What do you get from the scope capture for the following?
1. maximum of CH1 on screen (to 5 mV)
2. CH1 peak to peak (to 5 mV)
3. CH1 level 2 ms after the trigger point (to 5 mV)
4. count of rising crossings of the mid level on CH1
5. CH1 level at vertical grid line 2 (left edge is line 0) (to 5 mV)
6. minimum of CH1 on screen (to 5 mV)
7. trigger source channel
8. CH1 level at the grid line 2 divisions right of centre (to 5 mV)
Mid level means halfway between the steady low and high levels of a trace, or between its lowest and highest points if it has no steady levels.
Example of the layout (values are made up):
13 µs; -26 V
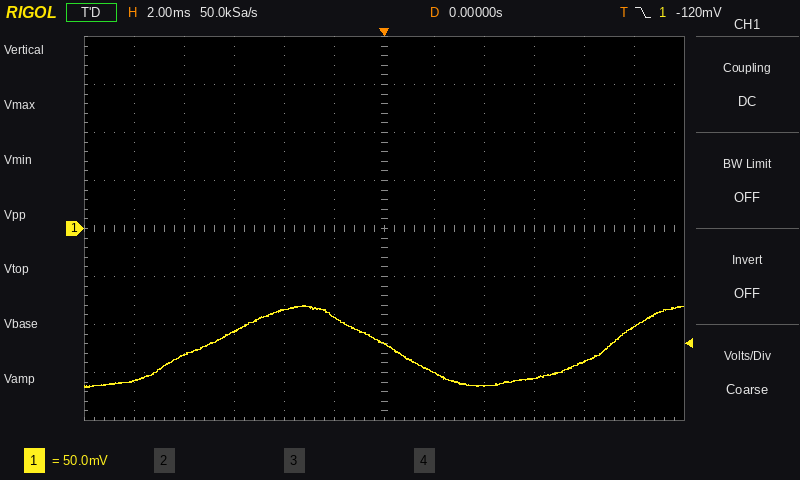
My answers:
-80 mV; 85 mV; -150 mV; 2; -130 mV; -165 mV; CH1; -165 mV
